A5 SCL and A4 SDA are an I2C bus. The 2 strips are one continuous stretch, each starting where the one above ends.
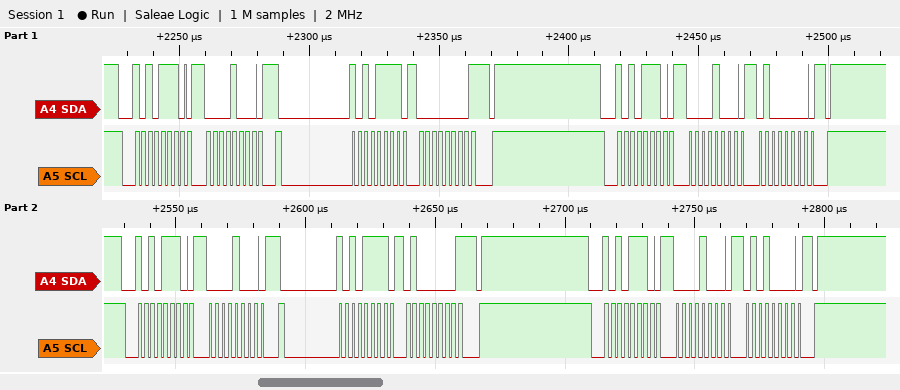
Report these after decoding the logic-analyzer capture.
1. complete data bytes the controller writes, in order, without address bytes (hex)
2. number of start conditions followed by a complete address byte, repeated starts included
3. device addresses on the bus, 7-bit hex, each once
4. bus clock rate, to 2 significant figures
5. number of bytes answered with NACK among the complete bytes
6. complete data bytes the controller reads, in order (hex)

08 08 40 08 08 50
6
0x57
400 kHz
2
00 40
